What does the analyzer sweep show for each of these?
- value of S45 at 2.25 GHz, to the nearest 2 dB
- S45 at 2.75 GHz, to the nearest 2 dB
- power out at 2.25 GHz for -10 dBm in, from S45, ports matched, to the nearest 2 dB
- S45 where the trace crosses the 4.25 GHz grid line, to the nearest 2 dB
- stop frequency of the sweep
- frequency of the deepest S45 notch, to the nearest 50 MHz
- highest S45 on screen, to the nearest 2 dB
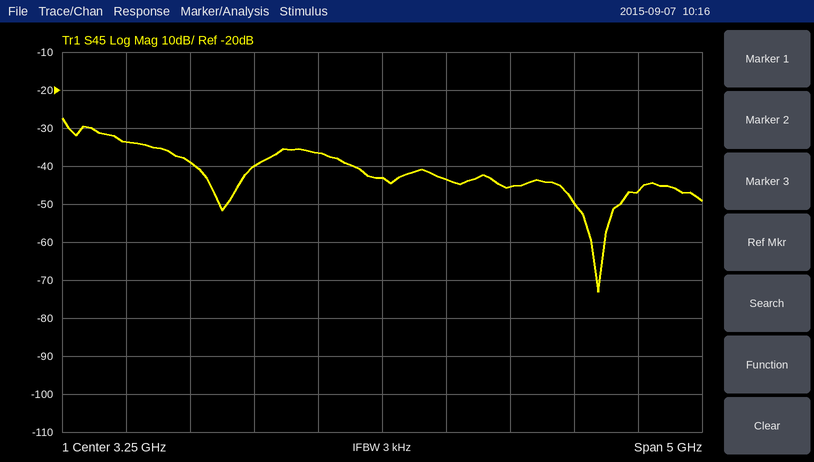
-40 dB
-36 dB
-50 dBm
-46 dB
5.75 GHz
4.95 GHz
-28 dB
